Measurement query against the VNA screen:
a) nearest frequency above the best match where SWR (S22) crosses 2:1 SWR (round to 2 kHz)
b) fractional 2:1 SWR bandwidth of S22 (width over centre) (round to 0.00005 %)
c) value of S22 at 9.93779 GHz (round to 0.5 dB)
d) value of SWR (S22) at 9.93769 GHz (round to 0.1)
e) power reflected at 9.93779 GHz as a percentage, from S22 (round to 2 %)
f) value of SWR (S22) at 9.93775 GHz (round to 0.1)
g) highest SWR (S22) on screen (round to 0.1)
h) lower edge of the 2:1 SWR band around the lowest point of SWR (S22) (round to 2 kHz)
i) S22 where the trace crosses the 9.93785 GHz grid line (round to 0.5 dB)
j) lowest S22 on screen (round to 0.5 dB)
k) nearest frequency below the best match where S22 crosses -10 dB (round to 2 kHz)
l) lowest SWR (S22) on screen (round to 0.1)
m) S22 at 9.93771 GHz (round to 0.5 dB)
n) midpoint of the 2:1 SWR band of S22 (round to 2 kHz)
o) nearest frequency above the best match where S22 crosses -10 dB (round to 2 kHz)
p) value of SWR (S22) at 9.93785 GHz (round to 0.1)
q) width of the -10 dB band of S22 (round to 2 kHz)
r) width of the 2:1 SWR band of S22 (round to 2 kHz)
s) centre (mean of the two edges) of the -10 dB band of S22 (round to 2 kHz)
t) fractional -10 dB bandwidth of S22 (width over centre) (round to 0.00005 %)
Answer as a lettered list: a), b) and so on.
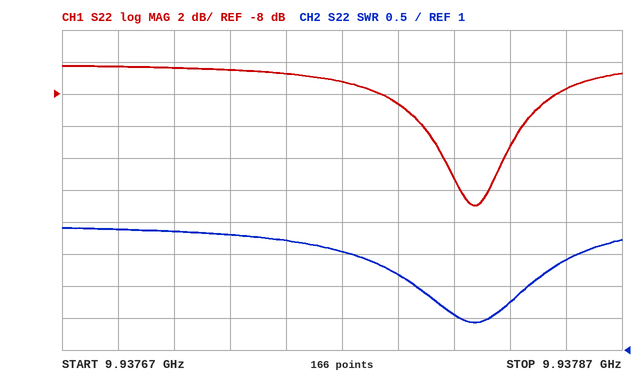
a) 9.937836 GHz
b) 0.00040 %
c) -8.5 dB
d) 2.9
e) 14 %
f) 2.7
g) 2.9
h) 9.937796 GHz
i) -7.5 dB
j) -15.0 dB
k) 9.937798 GHz
l) 1.4
m) -6.5 dB
n) 9.937816 GHz
o) 9.937834 GHz
p) 2.4
q) 36 kHz
r) 40 kHz
s) 9.937816 GHz
t) 0.00035 %
